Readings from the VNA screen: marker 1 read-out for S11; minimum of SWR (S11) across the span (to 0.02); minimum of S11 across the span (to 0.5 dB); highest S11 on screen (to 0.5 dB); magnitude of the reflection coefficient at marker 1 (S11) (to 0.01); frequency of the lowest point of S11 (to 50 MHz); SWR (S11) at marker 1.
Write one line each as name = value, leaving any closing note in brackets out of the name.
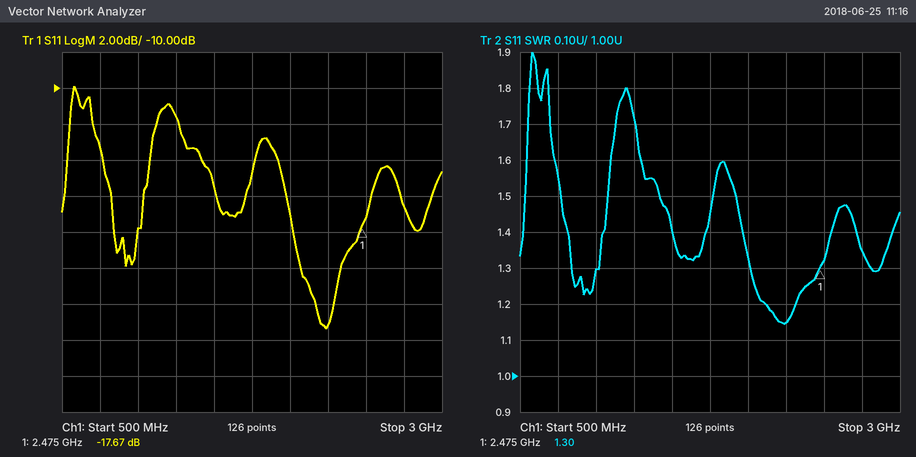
marker 1 read-out for S11 = -17.67 dB
minimum of SWR (S11) across the span = 1.14
minimum of S11 across the span = -23.5 dB
highest S11 on screen = -10.0 dB
magnitude of the reflection coefficient at marker 1 (S11) = 0.13
frequency of the lowest point of S11 = 2.25 GHz
SWR (S11) at marker 1 = 1.30
